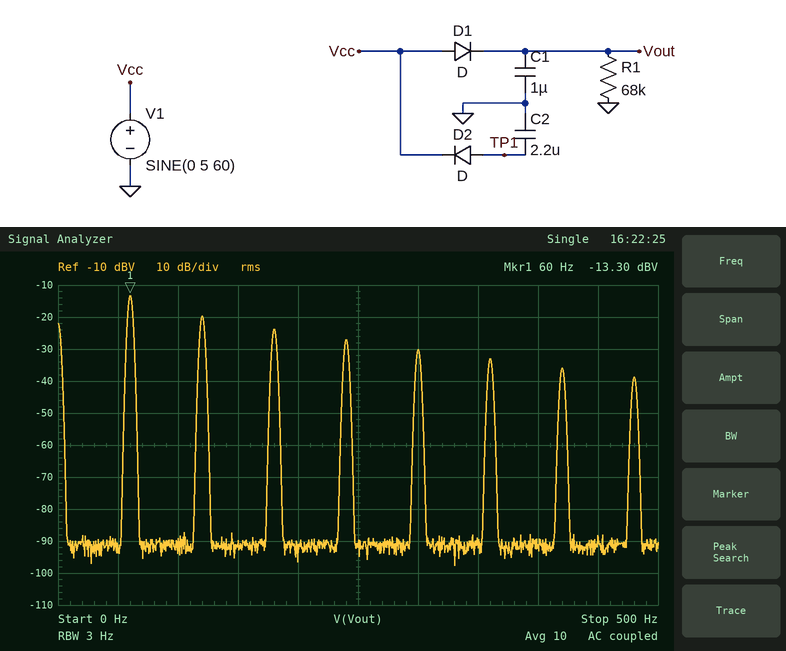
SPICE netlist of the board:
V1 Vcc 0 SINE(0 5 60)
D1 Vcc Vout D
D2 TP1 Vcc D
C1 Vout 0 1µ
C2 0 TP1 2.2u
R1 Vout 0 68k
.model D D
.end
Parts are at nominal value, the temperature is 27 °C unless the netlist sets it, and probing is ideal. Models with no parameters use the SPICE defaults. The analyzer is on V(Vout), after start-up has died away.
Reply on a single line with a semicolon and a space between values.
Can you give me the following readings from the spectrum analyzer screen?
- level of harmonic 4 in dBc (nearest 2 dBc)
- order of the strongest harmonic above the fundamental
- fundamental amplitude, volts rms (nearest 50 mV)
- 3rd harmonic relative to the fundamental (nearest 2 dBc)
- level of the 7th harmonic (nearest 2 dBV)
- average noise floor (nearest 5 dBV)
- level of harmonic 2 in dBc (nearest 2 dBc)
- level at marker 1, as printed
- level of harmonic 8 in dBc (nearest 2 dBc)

-14 dBc; 2; 200 mV; -10 dBc; -36 dBV; -90 dBV; -6 dBc; -13.30 dBV; -26 dBc
